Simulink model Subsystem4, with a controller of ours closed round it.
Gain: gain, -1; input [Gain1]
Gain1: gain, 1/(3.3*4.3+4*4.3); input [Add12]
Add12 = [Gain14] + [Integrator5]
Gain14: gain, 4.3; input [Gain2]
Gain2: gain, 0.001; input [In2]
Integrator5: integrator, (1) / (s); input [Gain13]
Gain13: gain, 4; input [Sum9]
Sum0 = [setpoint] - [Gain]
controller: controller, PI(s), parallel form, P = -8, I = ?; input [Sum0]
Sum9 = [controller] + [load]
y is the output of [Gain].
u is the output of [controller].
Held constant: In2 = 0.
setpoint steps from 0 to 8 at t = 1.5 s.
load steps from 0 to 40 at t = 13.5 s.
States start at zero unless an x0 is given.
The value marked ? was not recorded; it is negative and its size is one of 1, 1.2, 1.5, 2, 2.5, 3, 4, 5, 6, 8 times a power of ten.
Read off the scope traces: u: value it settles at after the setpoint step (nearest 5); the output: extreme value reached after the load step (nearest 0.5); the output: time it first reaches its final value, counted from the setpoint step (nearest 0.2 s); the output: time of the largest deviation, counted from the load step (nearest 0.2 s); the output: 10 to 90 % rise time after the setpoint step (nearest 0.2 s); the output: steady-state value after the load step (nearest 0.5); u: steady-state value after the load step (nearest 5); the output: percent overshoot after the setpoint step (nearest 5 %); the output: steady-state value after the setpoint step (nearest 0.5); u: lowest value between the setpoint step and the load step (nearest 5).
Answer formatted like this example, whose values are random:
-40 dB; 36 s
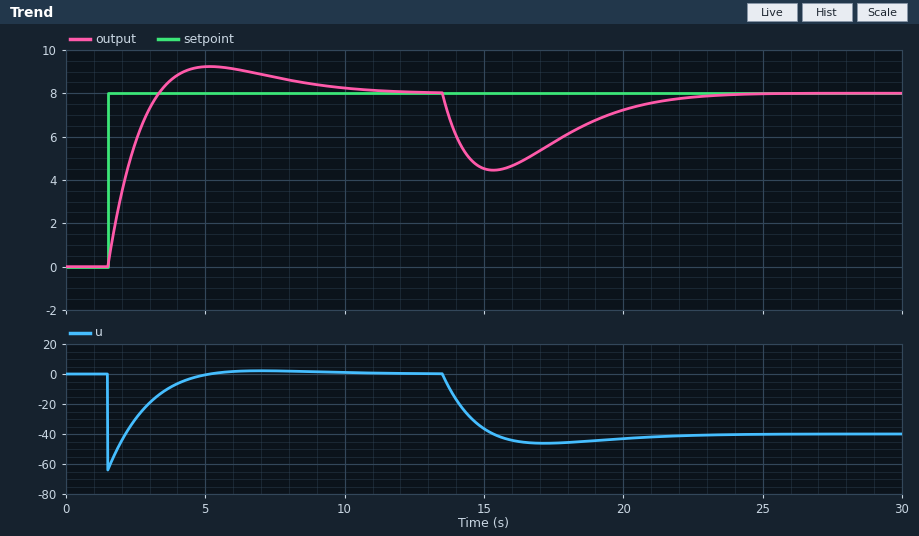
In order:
0; 4.5; 1.8 s; 1.8 s; 1.4 s; 8.0; -40; 15 %; 8.0; -65
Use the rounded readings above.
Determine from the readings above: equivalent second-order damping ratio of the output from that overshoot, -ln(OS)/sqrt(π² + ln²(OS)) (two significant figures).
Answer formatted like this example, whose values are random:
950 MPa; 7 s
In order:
0.52
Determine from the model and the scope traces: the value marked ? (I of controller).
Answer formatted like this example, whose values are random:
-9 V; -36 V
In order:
-2.5
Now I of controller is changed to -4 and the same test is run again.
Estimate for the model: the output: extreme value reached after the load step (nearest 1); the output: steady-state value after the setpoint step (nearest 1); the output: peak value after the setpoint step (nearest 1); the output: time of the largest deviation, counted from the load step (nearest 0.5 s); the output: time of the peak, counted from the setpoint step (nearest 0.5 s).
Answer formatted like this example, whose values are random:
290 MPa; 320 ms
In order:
5; 8; 10; 1.5 s; 3.0 s
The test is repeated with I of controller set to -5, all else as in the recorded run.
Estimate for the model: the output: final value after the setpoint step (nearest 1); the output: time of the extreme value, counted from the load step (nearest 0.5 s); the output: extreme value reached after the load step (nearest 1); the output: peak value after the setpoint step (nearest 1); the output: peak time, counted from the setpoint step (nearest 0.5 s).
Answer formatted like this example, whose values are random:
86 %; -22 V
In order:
8; 1.5 s; 5; 10; 3.0 s
